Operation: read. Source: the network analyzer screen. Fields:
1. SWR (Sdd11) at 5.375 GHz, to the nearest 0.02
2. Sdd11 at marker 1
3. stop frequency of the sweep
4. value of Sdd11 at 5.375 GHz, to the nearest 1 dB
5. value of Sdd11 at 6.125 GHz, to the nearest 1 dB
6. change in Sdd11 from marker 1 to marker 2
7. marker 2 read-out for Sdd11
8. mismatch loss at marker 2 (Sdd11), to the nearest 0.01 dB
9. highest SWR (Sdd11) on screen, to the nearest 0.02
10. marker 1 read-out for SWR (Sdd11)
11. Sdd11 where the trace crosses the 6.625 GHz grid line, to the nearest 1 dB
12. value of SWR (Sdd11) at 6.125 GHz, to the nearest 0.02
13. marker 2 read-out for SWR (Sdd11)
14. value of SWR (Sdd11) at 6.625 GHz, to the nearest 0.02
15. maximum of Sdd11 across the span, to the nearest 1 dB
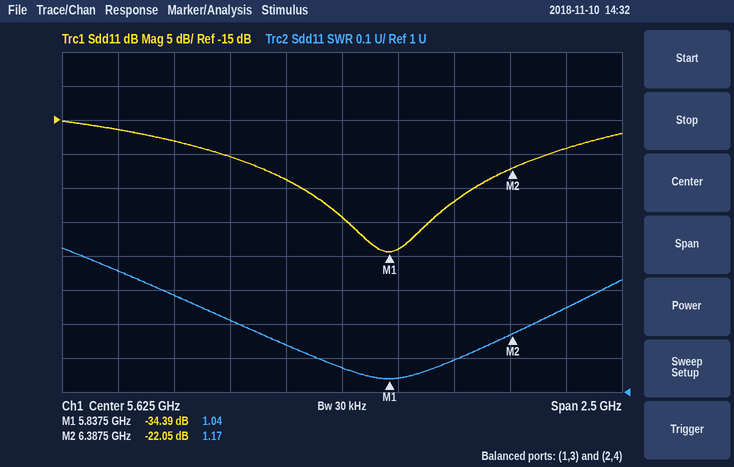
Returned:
1.14
-34.39 dB
6.875 GHz
-24 dB
-27 dB
12.34 dB
-22.05 dB
0.03 dB
1.42
1.04
-19 dB
1.10
1.17
1.24
-15 dB
